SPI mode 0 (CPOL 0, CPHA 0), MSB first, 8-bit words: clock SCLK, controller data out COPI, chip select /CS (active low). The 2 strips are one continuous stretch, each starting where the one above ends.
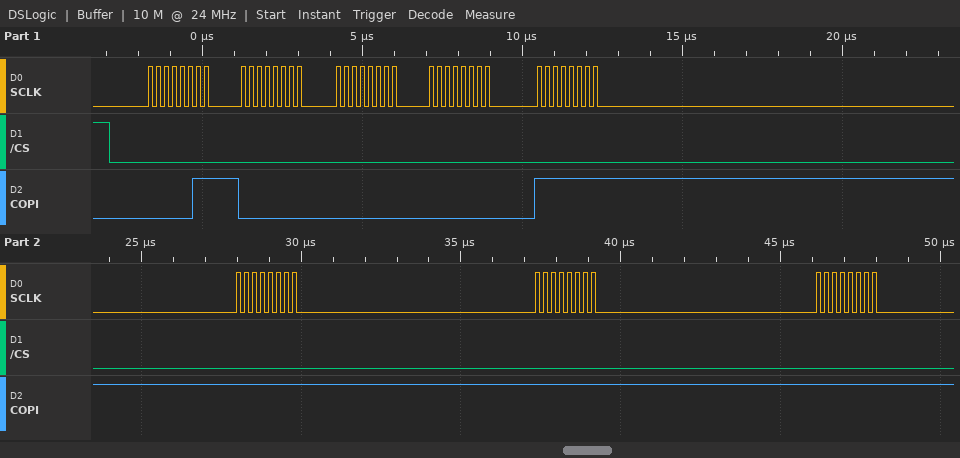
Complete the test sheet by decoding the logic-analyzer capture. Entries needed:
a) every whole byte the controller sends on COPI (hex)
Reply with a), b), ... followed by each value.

a) 0x03 0x00 0x00 0x00 0xFF 0xFF 0xFF 0xFF
